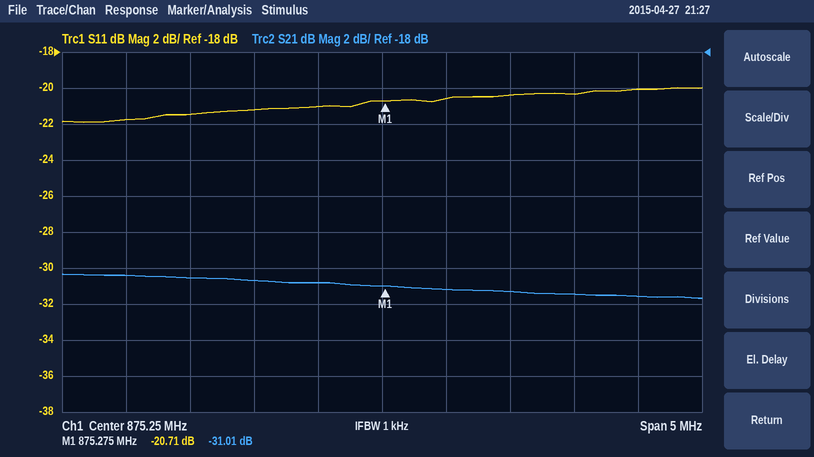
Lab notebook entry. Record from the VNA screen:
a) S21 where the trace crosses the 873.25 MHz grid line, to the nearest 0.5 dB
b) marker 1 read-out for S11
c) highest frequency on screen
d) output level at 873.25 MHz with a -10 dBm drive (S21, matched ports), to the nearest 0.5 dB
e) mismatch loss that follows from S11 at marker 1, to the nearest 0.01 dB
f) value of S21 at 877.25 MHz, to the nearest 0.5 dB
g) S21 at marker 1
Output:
-30.5 dB
-20.71 dB
877.75 MHz
-40.5 dBm
0.04 dB
-31.5 dB
-31.01 dB
